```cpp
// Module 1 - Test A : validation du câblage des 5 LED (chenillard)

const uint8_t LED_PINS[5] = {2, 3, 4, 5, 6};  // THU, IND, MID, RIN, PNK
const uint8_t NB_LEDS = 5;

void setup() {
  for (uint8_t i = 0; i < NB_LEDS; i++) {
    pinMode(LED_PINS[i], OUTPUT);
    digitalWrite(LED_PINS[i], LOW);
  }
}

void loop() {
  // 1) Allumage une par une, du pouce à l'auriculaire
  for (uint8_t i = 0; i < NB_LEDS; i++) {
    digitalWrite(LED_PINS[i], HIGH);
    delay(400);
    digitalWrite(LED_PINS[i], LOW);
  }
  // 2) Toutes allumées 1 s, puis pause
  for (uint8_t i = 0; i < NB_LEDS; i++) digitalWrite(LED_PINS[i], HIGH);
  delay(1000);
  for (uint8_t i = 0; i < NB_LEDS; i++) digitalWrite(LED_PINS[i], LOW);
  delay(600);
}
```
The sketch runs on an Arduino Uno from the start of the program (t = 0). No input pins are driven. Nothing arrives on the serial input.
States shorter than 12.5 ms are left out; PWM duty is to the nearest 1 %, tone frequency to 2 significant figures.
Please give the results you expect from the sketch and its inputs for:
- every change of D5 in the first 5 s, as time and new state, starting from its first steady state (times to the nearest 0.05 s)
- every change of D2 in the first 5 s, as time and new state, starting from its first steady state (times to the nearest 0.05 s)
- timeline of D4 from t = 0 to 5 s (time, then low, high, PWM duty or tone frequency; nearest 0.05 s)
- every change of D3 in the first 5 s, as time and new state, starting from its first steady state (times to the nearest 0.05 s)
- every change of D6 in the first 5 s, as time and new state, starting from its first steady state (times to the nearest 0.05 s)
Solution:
0 s low; 1.2 s high; 1.6 s low; 2 s high; 3 s low; 4.8 s high
0 s high; 0.4 s low; 2 s high; 3 s low; 3.6 s high; 4 s low
0 s low; 0.8 s high; 1.2 s low; 2 s high; 3 s low; 4.4 s high; 4.8 s low
0 s low; 0.4 s high; 0.8 s low; 2 s high; 3 s low; 4 s high; 4.4 s low
0 s low; 1.6 s high; 3 s low
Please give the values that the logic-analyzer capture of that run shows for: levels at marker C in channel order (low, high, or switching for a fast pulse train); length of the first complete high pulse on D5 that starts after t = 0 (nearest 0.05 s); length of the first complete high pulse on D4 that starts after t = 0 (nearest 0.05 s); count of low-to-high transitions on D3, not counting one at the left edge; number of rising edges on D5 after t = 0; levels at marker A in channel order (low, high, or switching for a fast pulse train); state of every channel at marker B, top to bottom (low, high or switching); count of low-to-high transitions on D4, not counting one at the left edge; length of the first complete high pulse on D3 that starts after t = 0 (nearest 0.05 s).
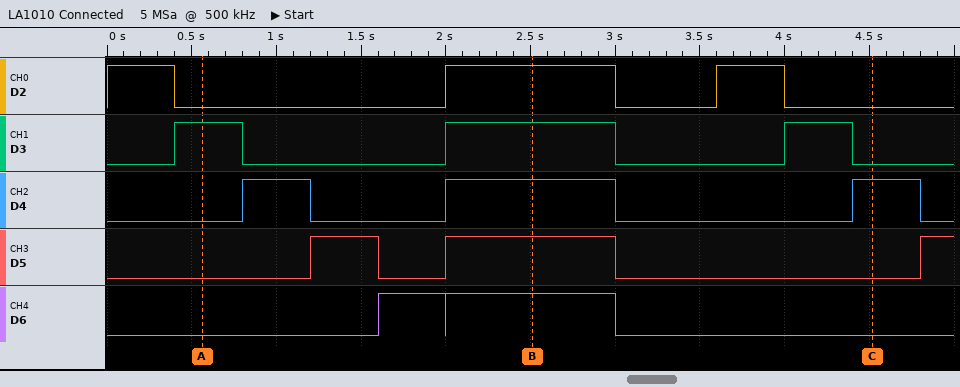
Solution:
D2 low, D3 low, D4 high, D5 low, D6 low
0.40 s
0.40 s
3
3
D2 low, D3 high, D4 low, D5 low, D6 low
D2 high, D3 high, D4 high, D5 high, D6 high
3
0.40 s
